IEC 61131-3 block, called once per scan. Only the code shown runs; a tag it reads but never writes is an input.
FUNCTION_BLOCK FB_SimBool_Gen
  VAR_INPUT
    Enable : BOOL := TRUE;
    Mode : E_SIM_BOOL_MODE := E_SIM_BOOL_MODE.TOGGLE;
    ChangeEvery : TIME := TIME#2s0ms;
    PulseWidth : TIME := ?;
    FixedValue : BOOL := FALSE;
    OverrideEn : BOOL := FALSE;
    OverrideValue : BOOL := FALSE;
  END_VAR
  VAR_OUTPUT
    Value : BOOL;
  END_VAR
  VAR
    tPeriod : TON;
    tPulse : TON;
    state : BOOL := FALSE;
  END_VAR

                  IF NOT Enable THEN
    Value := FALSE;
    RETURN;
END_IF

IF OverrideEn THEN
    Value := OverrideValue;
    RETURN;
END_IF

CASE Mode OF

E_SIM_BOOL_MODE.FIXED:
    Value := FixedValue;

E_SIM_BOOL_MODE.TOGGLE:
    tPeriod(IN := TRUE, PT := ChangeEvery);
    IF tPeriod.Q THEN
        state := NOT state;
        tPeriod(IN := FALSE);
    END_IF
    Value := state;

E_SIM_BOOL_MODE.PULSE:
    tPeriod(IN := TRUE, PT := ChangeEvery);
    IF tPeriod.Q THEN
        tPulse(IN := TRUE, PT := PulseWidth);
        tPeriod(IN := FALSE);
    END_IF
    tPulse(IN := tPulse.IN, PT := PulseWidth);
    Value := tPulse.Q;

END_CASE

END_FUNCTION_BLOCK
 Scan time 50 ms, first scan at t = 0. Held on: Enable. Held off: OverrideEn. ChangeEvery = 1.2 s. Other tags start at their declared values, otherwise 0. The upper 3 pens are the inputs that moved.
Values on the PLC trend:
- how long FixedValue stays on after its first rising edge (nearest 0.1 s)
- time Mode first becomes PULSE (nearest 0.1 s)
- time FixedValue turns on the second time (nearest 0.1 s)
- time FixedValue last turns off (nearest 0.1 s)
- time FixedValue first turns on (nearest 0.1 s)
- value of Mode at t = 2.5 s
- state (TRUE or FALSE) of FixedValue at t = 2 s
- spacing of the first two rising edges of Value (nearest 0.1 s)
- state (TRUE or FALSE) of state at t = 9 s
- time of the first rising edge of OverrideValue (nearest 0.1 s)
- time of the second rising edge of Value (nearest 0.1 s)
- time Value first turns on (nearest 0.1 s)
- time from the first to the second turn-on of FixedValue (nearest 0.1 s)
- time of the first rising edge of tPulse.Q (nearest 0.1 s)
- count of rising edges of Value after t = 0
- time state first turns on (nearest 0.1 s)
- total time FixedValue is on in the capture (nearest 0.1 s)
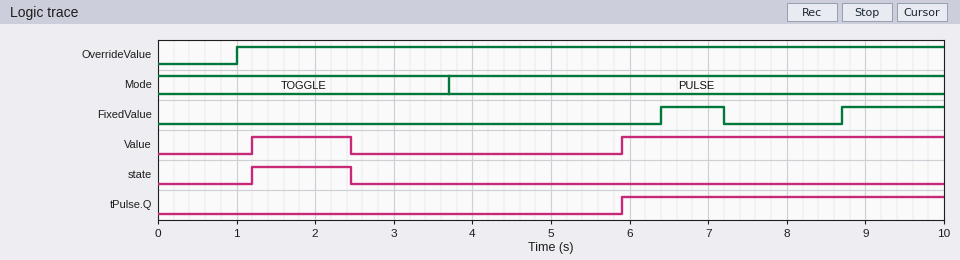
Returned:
0.8 s
3.7 s
8.7 s
7.2 s
6.4 s
TOGGLE
FALSE
4.7 s
FALSE
1.0 s
5.9 s
1.2 s
2.3 s
5.9 s
2
1.2 s
2.1 s
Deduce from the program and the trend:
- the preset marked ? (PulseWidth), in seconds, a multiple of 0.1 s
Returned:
2.2 s
